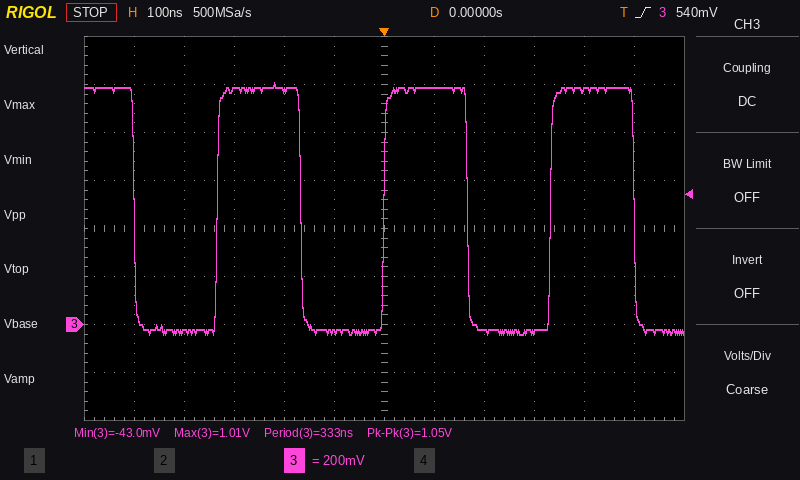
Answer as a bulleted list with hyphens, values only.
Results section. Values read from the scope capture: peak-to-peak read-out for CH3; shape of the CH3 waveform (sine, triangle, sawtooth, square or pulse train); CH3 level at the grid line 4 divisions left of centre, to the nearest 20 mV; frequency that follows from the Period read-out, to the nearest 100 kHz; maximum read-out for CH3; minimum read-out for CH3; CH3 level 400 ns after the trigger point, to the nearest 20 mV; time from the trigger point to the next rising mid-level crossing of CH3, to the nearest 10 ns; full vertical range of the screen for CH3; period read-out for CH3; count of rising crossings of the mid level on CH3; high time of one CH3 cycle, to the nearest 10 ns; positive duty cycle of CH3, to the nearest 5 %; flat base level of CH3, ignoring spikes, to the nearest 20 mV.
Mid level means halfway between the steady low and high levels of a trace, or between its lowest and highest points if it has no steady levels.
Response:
- 1.05 V
- square
- -40 mV
- 3.0 MHz
- 1.01 V
- -43.0 mV
- 980 mV
- 330 ns
- 1.6 V
- 333 ns
- 3
- 170 ns
- 50 %
- -20 mV
